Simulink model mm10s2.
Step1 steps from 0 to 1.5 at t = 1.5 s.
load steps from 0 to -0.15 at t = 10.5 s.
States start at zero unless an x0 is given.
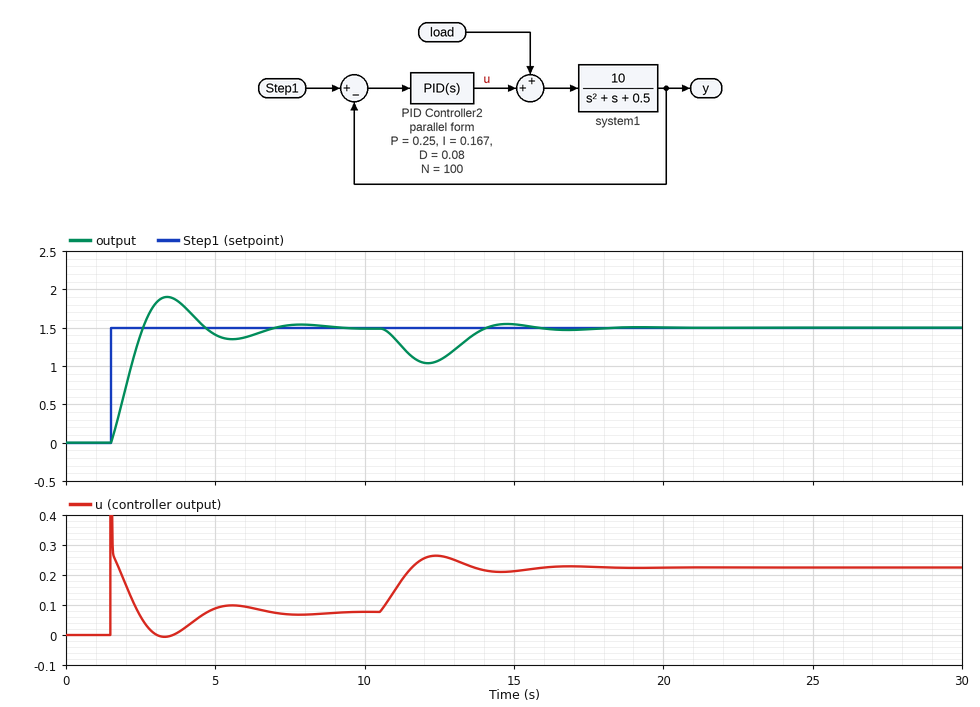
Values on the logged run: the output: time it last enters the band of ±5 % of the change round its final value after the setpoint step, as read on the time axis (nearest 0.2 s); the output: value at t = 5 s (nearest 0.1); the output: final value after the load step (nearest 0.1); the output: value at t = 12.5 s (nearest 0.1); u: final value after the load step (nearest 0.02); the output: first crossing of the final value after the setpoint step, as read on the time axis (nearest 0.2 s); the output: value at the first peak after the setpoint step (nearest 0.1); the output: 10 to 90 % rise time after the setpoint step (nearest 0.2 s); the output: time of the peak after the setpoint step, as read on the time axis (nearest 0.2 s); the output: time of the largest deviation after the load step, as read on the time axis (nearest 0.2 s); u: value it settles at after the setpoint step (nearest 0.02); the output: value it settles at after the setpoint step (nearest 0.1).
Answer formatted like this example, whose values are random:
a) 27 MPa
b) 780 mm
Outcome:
a) 6.4 s
b) 1.4
c) 1.5
d) 1.1
e) 0.22
f) 2.6 s
g) 1.9
h) 0.8 s
i) 3.4 s
j) 12.2 s
k) 0.08
l) 1.5
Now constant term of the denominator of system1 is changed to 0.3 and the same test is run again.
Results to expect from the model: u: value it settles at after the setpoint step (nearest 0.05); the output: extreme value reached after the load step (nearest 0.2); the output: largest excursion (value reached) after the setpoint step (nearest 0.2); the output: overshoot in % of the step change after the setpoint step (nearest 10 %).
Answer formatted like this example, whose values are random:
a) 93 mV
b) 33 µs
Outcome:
a) 0.05
b) 1.0
c) 2.0
d) 30 %
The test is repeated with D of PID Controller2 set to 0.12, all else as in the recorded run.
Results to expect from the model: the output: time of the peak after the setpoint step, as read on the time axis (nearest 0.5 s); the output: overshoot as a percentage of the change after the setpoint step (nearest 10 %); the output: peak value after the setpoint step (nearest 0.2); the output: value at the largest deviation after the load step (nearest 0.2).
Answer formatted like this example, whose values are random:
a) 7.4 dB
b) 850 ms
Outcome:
a) 3.5 s
b) 20 %
c) 1.8
d) 1.0
